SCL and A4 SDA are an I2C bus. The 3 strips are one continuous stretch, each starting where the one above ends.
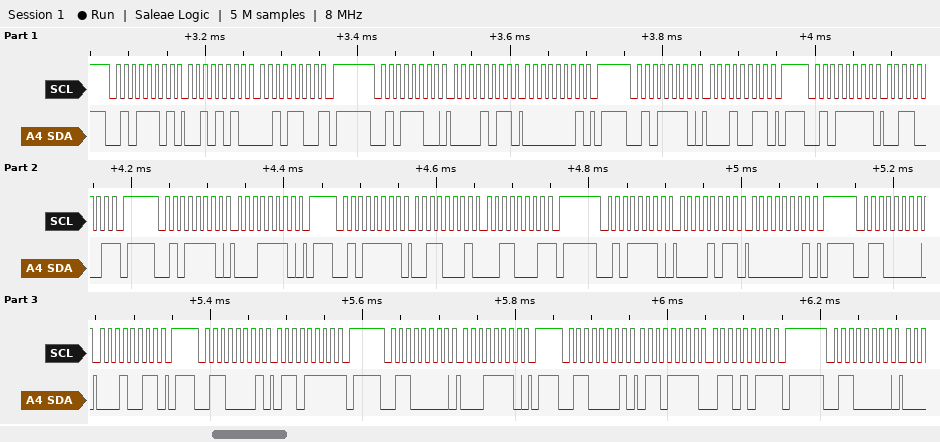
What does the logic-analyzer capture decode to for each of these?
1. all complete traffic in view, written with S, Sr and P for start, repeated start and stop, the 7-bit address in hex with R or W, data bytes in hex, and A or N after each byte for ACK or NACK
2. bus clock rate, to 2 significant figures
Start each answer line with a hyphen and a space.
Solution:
- S 2ER A 2A A 2C N P S 2EW A 0B A 01 A P S 2FW A 13 A P S 2FR A 31 N P S 2FW A 1E A P S 2FR A 31 A 31 N P S 2FW A 0B A 01 A P S 30W A 13 A P S 30R A 6F N P S 30W A 1E A P S 30R A 6F A 6B N P S 30W A
- 100 kHz
